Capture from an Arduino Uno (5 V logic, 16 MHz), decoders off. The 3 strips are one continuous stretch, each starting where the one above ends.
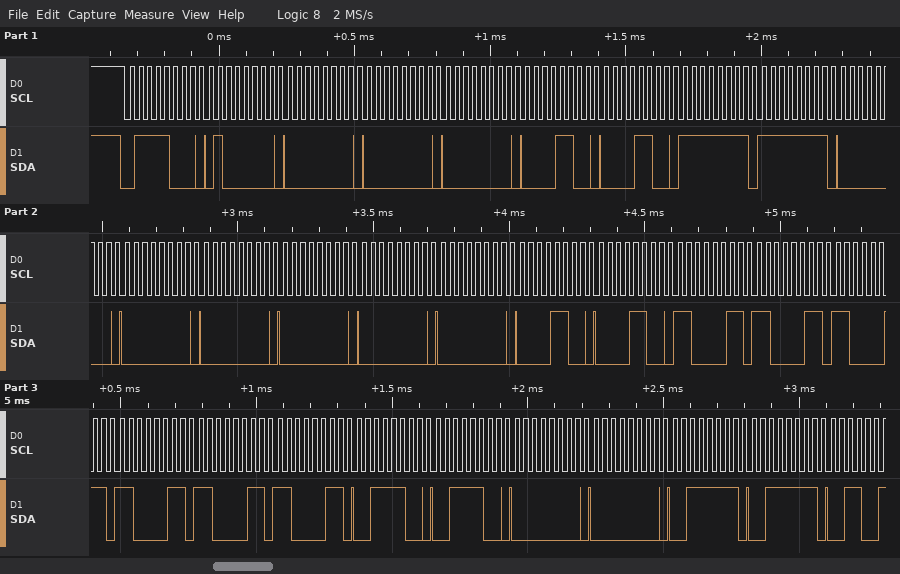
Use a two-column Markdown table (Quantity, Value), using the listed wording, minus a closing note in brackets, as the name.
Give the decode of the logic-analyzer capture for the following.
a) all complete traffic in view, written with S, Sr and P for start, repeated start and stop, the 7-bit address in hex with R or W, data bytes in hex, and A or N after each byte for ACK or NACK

| Quantity | Value |
|---|---|
| all complete traffic in view, written with S, Sr and P for start, repeated start and stop, the 7-bit address in hex with R or W, data bytes in hex, and A or N after each byte for ACK or NACK | S 3CW A 40 A 00 A 00 A 00 A 0C A 0C A FF A FF A 00 A 00 A 00 A 00 A 00 A 00 A 0C A 0C A C3 A C3 A C3 A C3 A C3 A C3 A 3C A 3C A 00 A 00 A 3F A 3F A |
